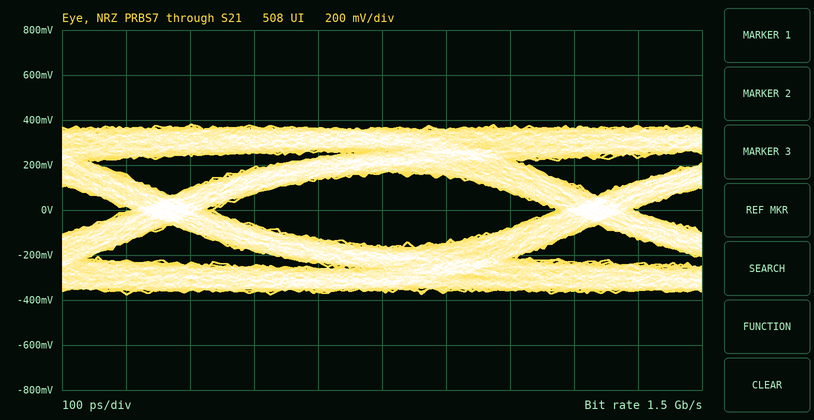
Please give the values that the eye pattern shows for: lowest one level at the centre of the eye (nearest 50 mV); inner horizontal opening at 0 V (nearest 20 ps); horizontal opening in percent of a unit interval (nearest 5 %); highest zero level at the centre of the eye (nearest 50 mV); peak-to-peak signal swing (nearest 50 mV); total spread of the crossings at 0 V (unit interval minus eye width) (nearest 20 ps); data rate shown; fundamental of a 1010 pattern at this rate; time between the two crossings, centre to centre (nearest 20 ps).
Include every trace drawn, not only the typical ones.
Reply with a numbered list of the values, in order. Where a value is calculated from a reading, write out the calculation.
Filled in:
1. 150 mV
2. 540 ps
3. 540 ps / 660 ps ≈ 81.8 %, so 80 % to the nearest 5 %
4. -150 mV
5. 750 mV
6. 120 ps
7. 1.5 Gb/s
8. 750 MHz
9. 660 ps
